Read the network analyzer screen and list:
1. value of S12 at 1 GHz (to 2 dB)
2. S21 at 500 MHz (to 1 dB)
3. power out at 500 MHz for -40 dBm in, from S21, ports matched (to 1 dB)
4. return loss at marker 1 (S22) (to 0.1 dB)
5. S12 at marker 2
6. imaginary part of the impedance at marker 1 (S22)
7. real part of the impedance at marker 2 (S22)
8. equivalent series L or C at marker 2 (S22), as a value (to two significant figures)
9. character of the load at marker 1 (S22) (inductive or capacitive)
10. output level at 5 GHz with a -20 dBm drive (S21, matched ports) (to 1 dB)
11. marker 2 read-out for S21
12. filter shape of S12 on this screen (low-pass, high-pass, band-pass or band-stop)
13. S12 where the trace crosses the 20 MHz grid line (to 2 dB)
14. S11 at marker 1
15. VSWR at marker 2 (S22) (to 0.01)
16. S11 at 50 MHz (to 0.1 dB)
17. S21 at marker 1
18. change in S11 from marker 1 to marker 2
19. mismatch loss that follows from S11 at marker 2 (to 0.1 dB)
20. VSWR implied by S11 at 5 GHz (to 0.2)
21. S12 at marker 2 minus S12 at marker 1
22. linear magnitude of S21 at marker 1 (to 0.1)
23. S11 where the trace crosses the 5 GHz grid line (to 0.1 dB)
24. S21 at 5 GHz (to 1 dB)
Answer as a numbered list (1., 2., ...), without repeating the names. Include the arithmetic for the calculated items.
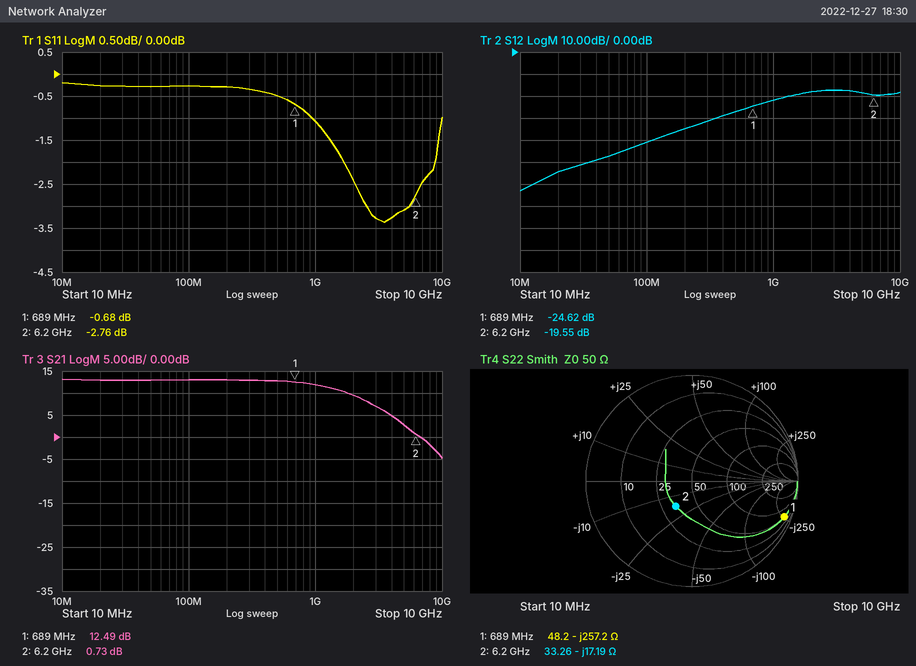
1. -22 dB
2. 13 dB
3. -40 dBm + (13 dB) = -27 dBm
4. 0.6 dB
5. -19.55 dB
6. -257.2 Ω
7. 33.26 Ω
8. C = 1/(2π × 6.2 GHz × 17.19 Ω) ≈ 1.5 pF
9. capacitive
10. -20 dBm + (3 dB) = -17 dBm
11. 0.73 dB
12. high-pass
13. -54 dB
14. -0.68 dB
15. 1.79
16. -0.3 dB
17. 12.49 dB
18. -2.76 − (-0.68) = -2.08 dB
19. −10 log10(1 − 10^(-2.76/10)) ≈ 3.3 dB
20. |Γ| = 10^(-3.1/20) = 0.6998; VSWR = (1 + 0.6998)/(1 − 0.6998) ≈ 5.66, so 5.6 to the nearest 0.2
21. -19.55 − (-24.62) = 5.07 dB
22. 10^(12.49/20) ≈ 4.2
23. -3.1 dB
24. 3 dB
